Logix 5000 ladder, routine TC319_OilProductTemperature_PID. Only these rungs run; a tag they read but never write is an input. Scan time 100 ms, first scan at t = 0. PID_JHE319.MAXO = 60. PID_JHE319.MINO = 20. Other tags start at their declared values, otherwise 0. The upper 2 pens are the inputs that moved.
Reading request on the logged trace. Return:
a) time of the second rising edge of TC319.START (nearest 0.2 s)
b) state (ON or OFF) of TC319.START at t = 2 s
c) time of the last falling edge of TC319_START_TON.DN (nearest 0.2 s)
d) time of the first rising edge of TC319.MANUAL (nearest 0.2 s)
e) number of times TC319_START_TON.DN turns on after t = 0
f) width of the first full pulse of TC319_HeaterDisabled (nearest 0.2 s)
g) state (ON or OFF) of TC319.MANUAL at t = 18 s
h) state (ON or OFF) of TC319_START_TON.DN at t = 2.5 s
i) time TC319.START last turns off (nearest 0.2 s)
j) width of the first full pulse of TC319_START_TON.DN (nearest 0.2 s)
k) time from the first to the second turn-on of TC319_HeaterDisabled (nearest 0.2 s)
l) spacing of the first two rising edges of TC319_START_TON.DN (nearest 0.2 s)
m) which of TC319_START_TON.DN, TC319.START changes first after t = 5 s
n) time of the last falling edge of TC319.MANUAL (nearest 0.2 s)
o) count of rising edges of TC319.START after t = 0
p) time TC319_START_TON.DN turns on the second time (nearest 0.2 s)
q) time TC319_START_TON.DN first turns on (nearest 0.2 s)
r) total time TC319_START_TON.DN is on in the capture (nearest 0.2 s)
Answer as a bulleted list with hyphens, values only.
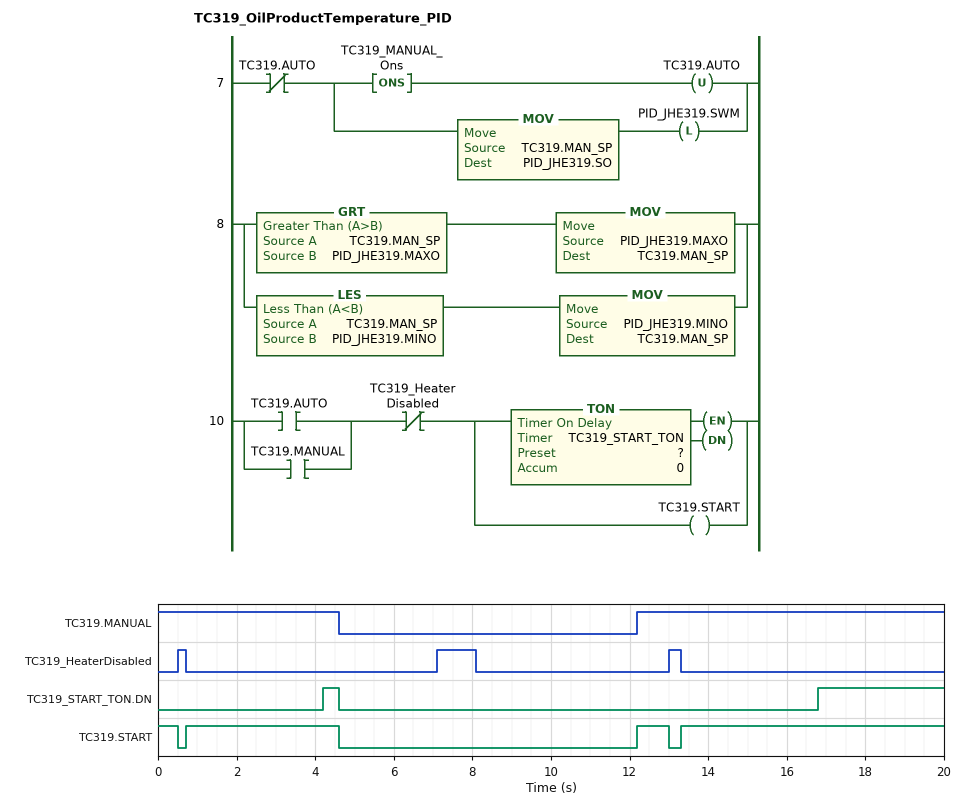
- 12.2 s
- ON
- 4.6 s
- 12.2 s
- 2
- 0.2 s
- ON
- OFF
- 13.0 s
- 0.4 s
- 6.6 s
- 12.6 s
- TC319.START
- 4.6 s
- 3
- 16.8 s
- 4.2 s
- 3.6 s
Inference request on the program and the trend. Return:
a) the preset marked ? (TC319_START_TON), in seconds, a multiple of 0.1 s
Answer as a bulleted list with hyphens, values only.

- 3.5 s
